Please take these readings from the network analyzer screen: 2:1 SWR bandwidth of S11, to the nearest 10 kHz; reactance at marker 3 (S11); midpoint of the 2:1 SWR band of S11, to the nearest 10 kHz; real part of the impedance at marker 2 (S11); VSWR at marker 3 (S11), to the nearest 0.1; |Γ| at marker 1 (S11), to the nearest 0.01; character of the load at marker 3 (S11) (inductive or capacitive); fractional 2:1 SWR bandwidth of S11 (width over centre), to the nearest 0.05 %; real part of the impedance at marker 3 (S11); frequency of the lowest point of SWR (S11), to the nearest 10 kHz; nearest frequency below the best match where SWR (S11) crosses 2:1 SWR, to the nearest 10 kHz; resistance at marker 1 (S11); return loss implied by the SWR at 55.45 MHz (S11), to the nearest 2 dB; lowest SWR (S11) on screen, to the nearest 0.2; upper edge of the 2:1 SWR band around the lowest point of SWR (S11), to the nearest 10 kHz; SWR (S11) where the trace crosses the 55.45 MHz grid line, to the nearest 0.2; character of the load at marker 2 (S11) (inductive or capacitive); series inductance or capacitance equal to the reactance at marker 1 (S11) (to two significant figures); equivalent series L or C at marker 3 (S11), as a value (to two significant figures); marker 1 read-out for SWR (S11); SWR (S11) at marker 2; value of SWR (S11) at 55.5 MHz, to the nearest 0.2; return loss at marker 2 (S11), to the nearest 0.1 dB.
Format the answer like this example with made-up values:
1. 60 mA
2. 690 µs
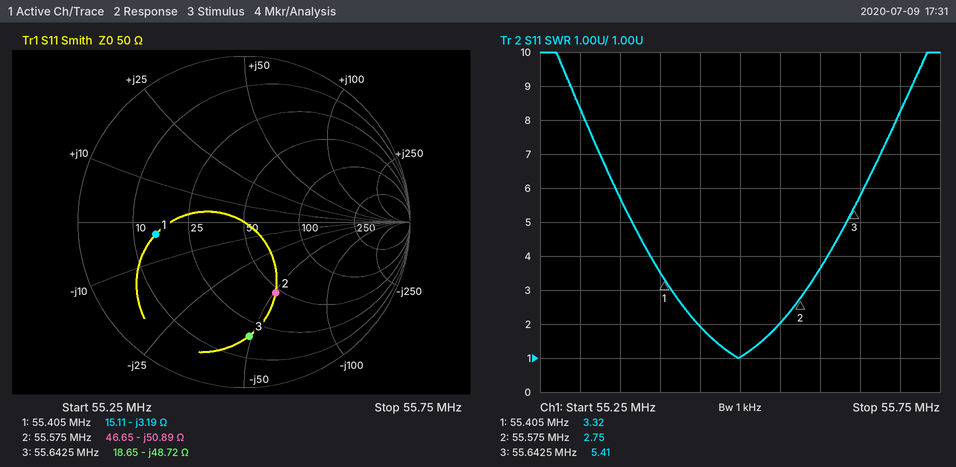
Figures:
1. 100 kHz
2. -48.72 Ω
3. 55.50 MHz
4. 46.65 Ω
5. 5.4
6. 0.54
7. capacitive
8. 0.20 %
9. 18.65 Ω
10. 55.50 MHz
11. 55.45 MHz
12. 15.11 Ω
13. 10 dB
14. 1.0
15. 55.55 MHz
16. 2.0
17. capacitive
18. 900 pF
19. 59 pF
20. 3.32
21. 2.75
22. 1.0
23. 6.6 dB
